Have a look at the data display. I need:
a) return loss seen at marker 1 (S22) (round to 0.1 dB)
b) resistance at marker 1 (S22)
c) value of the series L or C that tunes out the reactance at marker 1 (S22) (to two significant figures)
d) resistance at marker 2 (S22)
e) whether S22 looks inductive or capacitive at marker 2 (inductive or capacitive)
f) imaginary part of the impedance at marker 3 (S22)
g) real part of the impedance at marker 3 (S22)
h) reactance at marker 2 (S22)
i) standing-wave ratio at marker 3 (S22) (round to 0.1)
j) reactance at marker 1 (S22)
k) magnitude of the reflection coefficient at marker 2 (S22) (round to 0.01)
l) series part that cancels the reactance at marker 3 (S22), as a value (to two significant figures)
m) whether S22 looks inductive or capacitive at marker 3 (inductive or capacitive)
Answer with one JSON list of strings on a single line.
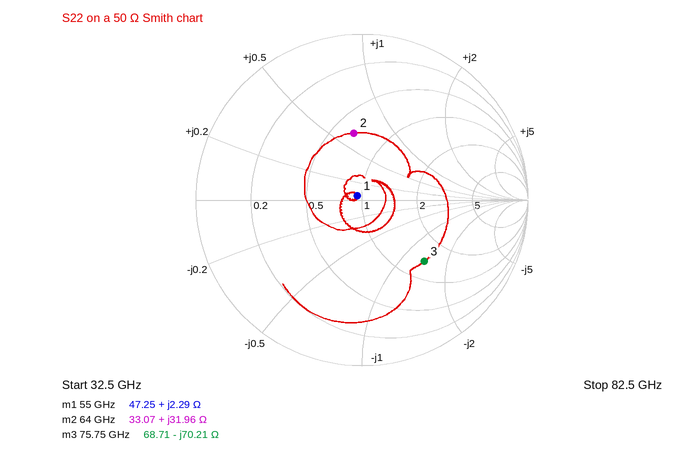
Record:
["28.7 dB", "47.25 Ω", "1.3 pF", "33.07 Ω", "inductive", "-70.21 Ω", "68.71 Ω", "+31.96 Ω", "3.2", "+2.29 Ω", "0.41", "150 pH", "capacitive"]
